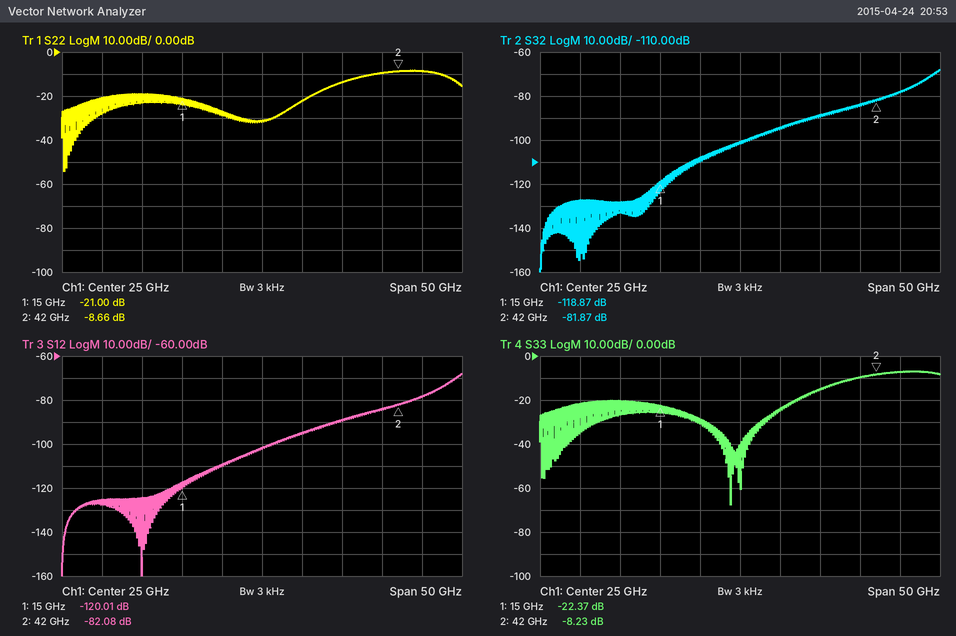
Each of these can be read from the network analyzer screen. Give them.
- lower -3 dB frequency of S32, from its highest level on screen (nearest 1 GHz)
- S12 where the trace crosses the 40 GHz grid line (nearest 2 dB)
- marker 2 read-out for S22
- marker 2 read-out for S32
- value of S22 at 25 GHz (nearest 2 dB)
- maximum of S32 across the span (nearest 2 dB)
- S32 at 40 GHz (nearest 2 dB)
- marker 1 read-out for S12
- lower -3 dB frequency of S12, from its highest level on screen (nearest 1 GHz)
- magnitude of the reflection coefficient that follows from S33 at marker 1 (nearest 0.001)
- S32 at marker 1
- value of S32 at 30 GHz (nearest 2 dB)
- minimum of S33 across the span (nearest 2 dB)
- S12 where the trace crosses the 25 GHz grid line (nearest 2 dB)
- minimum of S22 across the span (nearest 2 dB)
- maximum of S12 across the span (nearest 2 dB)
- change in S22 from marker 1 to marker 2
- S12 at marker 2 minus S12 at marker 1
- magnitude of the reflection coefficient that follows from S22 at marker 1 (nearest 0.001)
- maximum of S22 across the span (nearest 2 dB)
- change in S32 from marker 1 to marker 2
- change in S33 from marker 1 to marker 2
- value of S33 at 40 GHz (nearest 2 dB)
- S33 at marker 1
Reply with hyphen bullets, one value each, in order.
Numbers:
- 49 GHz
- -84 dB
- -8.66 dB
- -81.87 dB
- -32 dB
- -68 dB
- -84 dB
- -120.01 dB
- 49 GHz
- 0.076
- -118.87 dB
- -94 dB
- -68 dB
- -102 dB
- -54 dB
- -68 dB
- 12.34 dB
- 37.93 dB
- 0.089
- -8 dB
- 37.00 dB
- 14.14 dB
- -10 dB
- -22.37 dB
